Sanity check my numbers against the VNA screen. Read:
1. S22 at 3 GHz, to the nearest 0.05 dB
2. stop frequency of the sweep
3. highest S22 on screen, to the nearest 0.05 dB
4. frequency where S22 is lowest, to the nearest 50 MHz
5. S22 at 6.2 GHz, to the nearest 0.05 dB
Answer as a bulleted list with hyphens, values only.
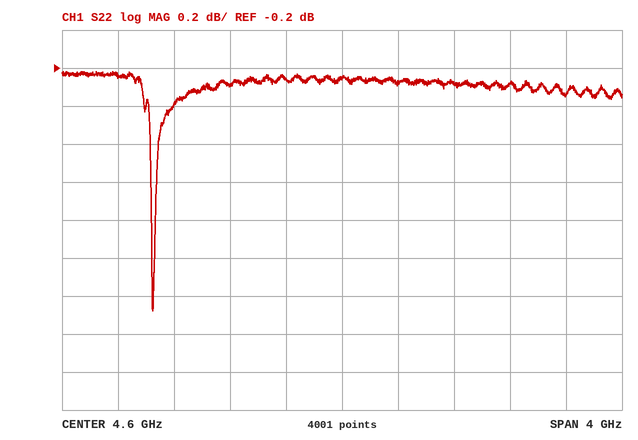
- -0.25 dB
- 6.6 GHz
- -0.20 dB
- 3.25 GHz
- -0.35 dB
